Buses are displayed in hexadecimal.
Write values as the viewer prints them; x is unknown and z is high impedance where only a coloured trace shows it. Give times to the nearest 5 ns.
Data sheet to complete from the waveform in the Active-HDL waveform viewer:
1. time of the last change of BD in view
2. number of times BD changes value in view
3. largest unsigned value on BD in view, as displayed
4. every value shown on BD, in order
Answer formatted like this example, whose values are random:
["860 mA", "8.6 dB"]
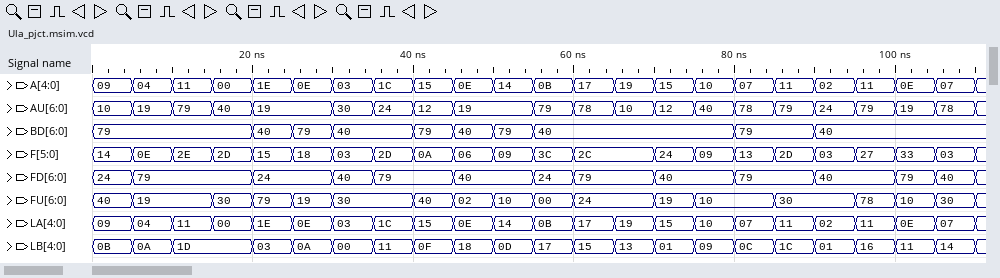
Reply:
["90 ns", "9", "79", "79, 40, 79, 40, 79, 40, 79, 40, 79, 40"]
